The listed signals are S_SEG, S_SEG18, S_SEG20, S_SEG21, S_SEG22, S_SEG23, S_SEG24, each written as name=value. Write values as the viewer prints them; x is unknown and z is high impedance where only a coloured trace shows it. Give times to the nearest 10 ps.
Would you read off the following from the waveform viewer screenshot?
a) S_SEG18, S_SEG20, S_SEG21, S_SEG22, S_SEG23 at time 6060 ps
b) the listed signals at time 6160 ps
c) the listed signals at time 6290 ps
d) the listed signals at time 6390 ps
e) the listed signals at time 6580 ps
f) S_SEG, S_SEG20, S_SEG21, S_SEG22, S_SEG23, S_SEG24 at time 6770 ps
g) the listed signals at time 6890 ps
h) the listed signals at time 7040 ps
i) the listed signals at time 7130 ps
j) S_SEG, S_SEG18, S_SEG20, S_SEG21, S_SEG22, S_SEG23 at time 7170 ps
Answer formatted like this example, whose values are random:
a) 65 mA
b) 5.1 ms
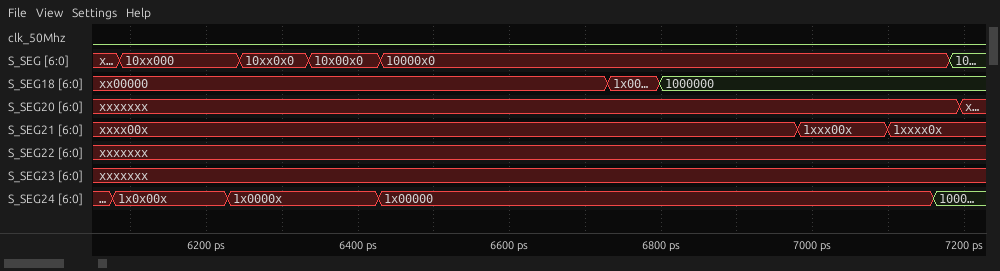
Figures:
a) S_SEG18=xx00000, S_SEG20=xxxxxxx, S_SEG21=xxxx00x, S_SEG22=xxxxxxx, S_SEG23=xxxxxxx
b) S_SEG=10xx000, S_SEG18=xx00000, S_SEG20=xxxxxxx, S_SEG21=xxxx00x, S_SEG22=xxxxxxx, S_SEG23=xxxxxxx, S_SEG24=1x0x00x
c) S_SEG=10xx0x0, S_SEG18=xx00000, S_SEG20=xxxxxxx, S_SEG21=xxxx00x, S_SEG22=xxxxxxx, S_SEG23=xxxxxxx, S_SEG24=1x0000x
d) S_SEG=10x00x0, S_SEG18=xx00000, S_SEG20=xxxxxxx, S_SEG21=xxxx00x, S_SEG22=xxxxxxx, S_SEG23=xxxxxxx, S_SEG24=1x0000x
e) S_SEG=10000x0, S_SEG18=xx00000, S_SEG20=xxxxxxx, S_SEG21=xxxx00x, S_SEG22=xxxxxxx, S_SEG23=xxxxxxx, S_SEG24=1x00000
f) S_SEG=10000x0, S_SEG20=xxxxxxx, S_SEG21=xxxx00x, S_SEG22=xxxxxxx, S_SEG23=xxxxxxx, S_SEG24=1x00000
g) S_SEG=10000x0, S_SEG18=1000000, S_SEG20=xxxxxxx, S_SEG21=xxxx00x, S_SEG22=xxxxxxx, S_SEG23=xxxxxxx, S_SEG24=1x00000
h) S_SEG=10000x0, S_SEG18=1000000, S_SEG20=xxxxxxx, S_SEG21=1xxx00x, S_SEG22=xxxxxxx, S_SEG23=xxxxxxx, S_SEG24=1x00000
i) S_SEG=10000x0, S_SEG18=1000000, S_SEG20=xxxxxxx, S_SEG21=1xxxx0x, S_SEG22=xxxxxxx, S_SEG23=xxxxxxx, S_SEG24=1x00000
j) S_SEG=10000x0, S_SEG18=1000000, S_SEG20=xxxxxxx, S_SEG21=1xxxx0x, S_SEG22=xxxxxxx, S_SEG23=xxxxxxx
